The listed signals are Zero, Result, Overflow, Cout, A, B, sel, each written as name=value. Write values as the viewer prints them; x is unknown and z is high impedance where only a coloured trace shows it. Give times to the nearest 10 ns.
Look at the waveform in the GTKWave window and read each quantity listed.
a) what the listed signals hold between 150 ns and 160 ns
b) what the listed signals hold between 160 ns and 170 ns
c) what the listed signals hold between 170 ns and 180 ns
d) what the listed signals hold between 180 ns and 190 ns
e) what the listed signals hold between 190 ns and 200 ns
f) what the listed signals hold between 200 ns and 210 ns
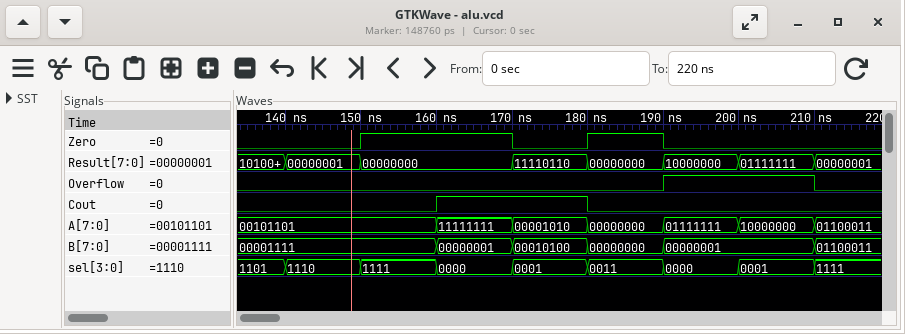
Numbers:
Zero=1, Result=00000000, Overflow=0, Cout=0, A=00101101, B=00001111, sel=1111
Zero=1, Result=00000000, Overflow=0, Cout=1, A=11111111, B=00000001, sel=0000
Zero=0, Result=11110110, Overflow=0, Cout=1, A=00001010, B=00010100, sel=0001
Zero=1, Result=00000000, Overflow=0, Cout=0, A=00000000, B=00000000, sel=0011
Zero=0, Result=10000000, Overflow=1, Cout=0, A=01111111, B=00000001, sel=0000
Zero=0, Result=01111111, Overflow=1, Cout=0, A=10000000, B=00000001, sel=0001
